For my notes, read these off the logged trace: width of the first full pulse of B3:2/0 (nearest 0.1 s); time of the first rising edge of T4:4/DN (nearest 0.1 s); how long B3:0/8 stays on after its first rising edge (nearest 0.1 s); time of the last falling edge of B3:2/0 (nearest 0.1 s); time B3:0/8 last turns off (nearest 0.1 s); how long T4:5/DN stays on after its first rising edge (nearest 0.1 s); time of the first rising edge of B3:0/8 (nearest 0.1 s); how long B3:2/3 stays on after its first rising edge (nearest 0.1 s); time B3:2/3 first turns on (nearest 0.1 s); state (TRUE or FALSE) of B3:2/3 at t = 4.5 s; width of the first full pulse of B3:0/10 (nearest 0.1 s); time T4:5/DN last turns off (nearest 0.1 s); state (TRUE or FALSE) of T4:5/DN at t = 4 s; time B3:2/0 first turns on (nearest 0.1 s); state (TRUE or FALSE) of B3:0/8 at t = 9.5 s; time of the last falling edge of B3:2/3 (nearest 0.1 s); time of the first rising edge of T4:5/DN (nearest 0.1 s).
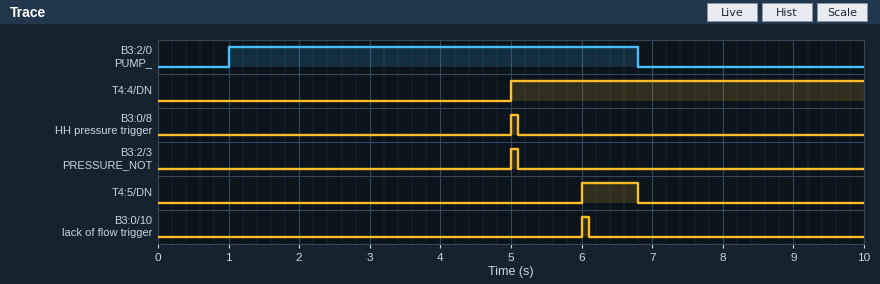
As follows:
5.8 s
5.0 s
0.1 s
6.8 s
5.1 s
0.8 s
5.0 s
0.1 s
5.0 s
FALSE
0.1 s
6.8 s
FALSE
1.0 s
FALSE
5.1 s
6.0 s
